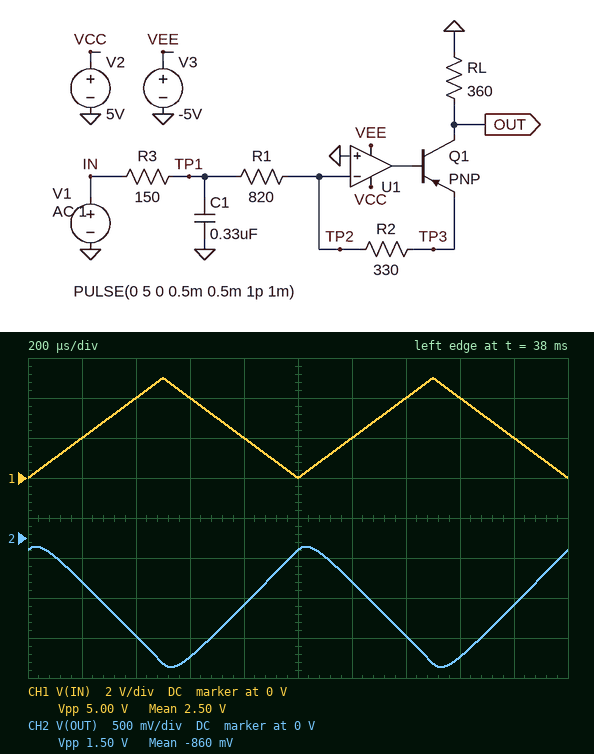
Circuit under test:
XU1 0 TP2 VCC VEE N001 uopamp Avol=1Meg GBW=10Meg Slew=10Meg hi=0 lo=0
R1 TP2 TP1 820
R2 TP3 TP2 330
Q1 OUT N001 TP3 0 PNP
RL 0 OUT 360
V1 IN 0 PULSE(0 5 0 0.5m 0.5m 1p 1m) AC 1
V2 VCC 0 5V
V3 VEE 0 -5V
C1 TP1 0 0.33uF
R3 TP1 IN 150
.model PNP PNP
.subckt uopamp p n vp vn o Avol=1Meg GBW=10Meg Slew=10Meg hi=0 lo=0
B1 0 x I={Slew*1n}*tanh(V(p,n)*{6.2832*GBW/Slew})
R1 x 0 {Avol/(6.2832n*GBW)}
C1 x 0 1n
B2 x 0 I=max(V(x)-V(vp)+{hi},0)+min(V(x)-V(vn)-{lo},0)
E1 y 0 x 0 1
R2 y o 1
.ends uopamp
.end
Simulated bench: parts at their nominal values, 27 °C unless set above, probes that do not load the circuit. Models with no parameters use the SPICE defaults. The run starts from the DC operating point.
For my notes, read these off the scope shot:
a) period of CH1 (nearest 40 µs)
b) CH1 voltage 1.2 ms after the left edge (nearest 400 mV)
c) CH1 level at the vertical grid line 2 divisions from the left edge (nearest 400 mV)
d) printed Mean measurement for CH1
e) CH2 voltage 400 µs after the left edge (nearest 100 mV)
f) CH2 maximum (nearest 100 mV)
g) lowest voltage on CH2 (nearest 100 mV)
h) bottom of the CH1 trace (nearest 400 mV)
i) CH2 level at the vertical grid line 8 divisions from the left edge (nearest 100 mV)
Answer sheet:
1.00 ms
2.0 V
4.0 V
2.50 V
-1.2 V
-100 mV
-1.6 V
0 V
-1.5 V
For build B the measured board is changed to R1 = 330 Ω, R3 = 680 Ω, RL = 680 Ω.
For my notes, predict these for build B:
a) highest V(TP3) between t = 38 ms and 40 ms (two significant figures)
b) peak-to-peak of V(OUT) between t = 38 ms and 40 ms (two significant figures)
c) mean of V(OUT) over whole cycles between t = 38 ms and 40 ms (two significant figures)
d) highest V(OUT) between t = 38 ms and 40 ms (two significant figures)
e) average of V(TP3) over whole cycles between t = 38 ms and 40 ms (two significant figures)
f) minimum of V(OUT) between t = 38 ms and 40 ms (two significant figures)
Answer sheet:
-170 mV
1.3 V
-830 mV
-180 mV
-820 mV
-1.5 V
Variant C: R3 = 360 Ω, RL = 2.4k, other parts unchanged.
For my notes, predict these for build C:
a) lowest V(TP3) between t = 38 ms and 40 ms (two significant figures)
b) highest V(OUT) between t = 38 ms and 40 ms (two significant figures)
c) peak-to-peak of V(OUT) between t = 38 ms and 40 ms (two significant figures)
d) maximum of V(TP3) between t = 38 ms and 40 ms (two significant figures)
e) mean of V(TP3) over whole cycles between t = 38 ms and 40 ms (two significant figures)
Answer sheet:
-1.2 V
-180 mV
1.1 V
-160 mV
-700 mV
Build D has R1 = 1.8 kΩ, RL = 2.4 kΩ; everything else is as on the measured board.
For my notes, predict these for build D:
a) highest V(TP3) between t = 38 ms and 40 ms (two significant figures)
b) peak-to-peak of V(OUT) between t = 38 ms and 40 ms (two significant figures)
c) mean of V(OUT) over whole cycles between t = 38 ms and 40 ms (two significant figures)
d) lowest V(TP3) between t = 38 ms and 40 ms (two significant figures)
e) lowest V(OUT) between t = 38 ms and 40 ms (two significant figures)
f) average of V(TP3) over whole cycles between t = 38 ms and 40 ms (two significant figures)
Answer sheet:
-54 mV
740 mV
-440 mV
-790 mV
-810 mV
-420 mV
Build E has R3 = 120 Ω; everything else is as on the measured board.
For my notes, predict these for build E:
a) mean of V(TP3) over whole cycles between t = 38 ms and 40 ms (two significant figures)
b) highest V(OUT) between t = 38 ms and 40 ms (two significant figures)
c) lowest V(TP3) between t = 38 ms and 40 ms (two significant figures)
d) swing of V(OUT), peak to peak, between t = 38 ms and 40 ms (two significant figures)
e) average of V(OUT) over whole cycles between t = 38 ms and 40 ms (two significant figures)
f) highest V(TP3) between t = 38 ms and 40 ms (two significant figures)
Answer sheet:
-880 mV
-94 mV
-1.7 V
1.6 V
-890 mV
-84 mV
